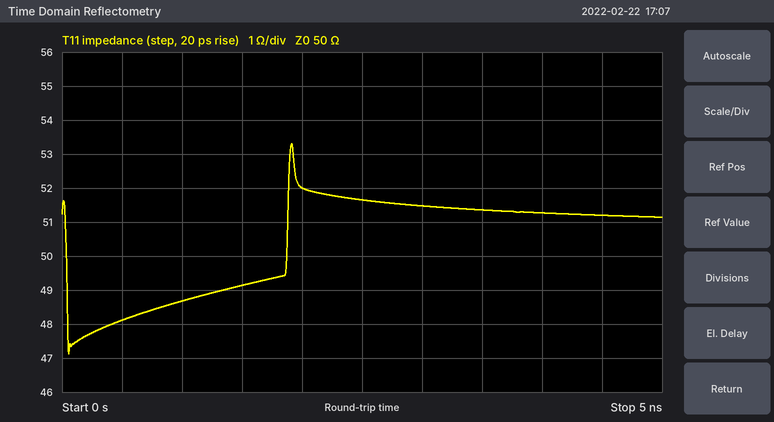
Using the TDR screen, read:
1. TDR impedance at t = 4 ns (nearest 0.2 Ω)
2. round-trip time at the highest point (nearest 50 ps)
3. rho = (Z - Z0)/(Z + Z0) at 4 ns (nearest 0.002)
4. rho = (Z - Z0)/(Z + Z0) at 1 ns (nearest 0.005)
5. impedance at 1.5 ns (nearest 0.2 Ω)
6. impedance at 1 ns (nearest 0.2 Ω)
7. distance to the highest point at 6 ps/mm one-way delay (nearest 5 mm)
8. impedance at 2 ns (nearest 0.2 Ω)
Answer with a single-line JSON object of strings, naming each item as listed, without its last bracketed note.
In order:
{"TDR impedance at t = 4 ns": "51.2 Ω", "round-trip time at the highest point": "1.90 ns", "rho = (Z - Z0)/(Z + Z0) at 4 ns": "+0.012", "rho = (Z - Z0)/(Z + Z0) at 1 ns": "-0.015", "impedance at 1.5 ns": "49.2 Ω", "impedance at 1 ns": "48.6 Ω", "distance to the highest point at 6 ps/mm one-way delay": "160 mm", "impedance at 2 ns": "52.0 Ω"}
